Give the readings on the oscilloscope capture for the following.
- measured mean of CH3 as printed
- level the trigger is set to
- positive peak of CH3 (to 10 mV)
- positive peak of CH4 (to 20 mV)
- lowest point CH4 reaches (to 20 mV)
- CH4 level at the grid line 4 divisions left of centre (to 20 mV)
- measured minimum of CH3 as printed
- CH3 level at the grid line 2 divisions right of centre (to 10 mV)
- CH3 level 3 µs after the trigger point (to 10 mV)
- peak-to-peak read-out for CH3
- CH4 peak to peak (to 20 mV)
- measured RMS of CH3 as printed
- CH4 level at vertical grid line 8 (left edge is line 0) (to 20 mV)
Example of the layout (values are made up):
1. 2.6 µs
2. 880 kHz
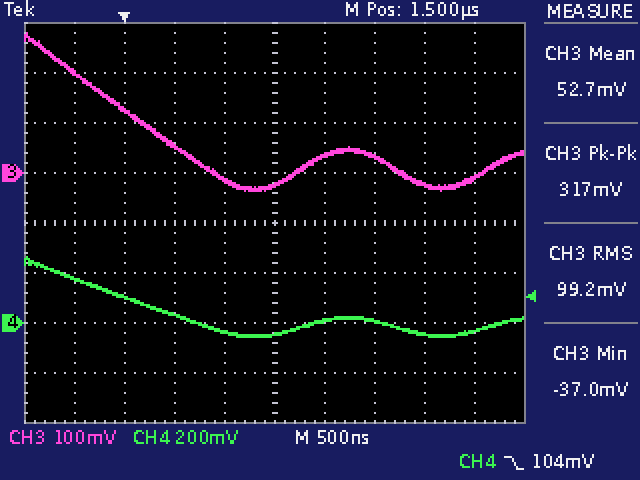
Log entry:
1. 52.7 mV
2. 104 mV
3. 280 mV
4. 260 mV
5. -60 mV
6. 180 mV
7. -37.0 mV
8. 30 mV
9. -20 mV
10. 317 mV
11. 320 mV
12. 99.2 mV
13. -40 mV
